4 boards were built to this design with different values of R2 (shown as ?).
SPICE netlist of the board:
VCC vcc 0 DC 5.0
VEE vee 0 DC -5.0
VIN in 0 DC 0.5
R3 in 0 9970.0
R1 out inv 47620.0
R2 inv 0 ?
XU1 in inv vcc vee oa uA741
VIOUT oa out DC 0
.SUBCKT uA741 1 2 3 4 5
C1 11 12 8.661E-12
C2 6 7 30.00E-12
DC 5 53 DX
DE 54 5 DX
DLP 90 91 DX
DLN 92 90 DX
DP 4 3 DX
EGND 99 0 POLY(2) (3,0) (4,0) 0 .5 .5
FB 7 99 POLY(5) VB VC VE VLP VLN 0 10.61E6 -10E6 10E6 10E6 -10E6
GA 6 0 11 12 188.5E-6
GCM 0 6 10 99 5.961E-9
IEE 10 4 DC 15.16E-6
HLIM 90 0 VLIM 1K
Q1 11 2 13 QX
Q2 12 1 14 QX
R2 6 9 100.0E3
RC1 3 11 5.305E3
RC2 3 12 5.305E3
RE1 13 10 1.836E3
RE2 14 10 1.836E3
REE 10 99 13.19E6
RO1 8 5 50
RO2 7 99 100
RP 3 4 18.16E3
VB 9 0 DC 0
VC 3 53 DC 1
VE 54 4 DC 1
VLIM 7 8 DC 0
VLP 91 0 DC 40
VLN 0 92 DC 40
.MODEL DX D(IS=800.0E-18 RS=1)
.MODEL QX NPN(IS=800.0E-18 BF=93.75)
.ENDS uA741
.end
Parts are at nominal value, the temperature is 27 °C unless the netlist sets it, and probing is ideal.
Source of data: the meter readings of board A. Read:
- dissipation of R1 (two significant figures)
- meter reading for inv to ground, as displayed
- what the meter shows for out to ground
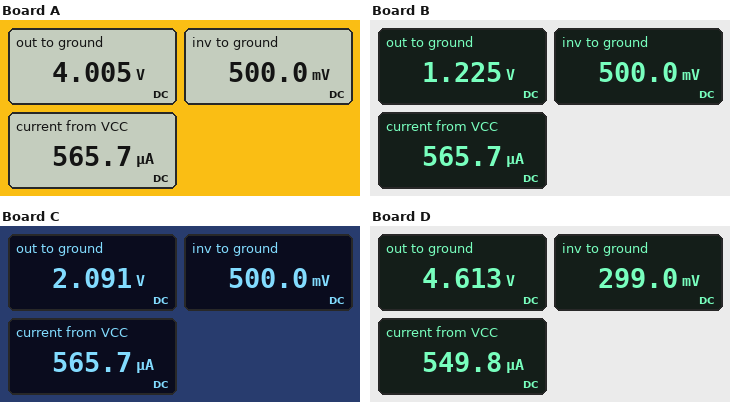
260 µW
500.0 mV
4.005 V
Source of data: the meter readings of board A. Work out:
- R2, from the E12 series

6.8 kΩ
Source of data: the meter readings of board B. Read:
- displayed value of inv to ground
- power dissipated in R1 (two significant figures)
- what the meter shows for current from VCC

500.0 mV
11 µW
565.7 µA
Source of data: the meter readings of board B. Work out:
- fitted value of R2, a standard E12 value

33 kΩ
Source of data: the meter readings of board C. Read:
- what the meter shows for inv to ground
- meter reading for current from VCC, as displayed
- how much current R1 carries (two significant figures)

500.0 mV
565.7 µA
33 µA
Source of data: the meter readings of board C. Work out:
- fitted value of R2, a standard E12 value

15 kΩ
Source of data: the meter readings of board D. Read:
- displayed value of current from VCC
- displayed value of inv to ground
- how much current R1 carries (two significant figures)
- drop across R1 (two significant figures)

549.8 µA
299.0 mV
91 µA
4.3 V
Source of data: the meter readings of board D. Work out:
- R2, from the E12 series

3.3 kΩ
